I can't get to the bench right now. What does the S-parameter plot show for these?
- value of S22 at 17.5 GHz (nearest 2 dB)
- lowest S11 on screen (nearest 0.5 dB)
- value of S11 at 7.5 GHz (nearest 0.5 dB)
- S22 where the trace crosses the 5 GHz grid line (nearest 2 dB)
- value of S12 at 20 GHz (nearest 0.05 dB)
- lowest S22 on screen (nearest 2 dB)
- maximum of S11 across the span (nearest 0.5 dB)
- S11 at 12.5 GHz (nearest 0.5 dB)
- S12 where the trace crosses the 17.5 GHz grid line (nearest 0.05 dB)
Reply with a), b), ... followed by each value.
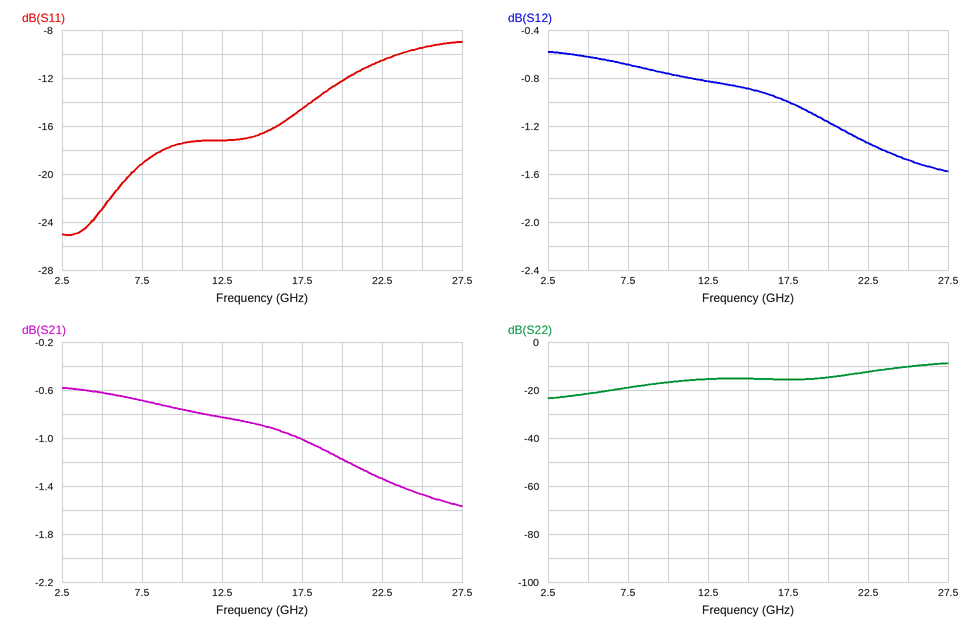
a) -16 dB
b) -25.0 dB
c) -19.0 dB
d) -22 dB
e) -1.15 dB
f) -24 dB
g) -9.0 dB
h) -17.0 dB
i) -1.00 dB
